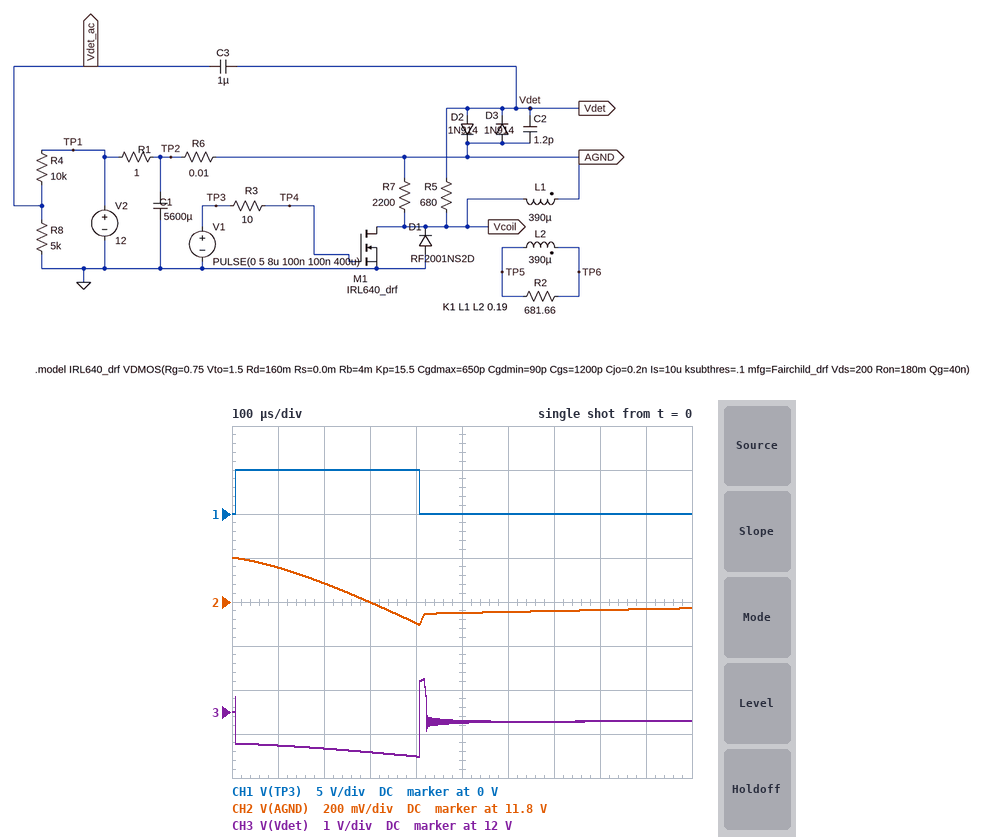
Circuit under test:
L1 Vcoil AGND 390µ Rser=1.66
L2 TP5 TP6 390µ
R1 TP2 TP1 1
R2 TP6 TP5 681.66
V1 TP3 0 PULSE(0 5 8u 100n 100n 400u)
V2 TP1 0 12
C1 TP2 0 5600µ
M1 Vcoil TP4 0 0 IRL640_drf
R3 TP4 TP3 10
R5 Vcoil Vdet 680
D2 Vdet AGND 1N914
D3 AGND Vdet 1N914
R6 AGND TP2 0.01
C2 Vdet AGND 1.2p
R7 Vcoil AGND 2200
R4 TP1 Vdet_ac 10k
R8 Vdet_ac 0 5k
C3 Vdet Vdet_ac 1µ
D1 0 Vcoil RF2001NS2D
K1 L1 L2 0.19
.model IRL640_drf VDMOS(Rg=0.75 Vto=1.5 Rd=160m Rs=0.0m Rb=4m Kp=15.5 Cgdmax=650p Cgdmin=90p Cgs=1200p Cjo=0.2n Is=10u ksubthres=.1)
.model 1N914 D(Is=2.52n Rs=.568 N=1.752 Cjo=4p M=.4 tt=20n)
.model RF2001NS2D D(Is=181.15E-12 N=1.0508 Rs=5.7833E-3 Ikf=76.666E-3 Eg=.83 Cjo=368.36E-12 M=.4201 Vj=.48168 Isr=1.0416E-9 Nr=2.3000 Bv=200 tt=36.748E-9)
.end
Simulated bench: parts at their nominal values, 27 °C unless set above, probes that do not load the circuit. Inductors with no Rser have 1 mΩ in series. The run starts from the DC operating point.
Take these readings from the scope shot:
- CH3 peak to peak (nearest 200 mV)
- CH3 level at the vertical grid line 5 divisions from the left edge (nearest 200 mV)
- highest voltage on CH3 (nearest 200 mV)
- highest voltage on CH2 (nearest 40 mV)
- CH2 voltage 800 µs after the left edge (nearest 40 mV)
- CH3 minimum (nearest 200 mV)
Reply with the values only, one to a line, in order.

1.8 V
11.8 V
12.8 V
12.00 V
11.76 V
11.0 V
